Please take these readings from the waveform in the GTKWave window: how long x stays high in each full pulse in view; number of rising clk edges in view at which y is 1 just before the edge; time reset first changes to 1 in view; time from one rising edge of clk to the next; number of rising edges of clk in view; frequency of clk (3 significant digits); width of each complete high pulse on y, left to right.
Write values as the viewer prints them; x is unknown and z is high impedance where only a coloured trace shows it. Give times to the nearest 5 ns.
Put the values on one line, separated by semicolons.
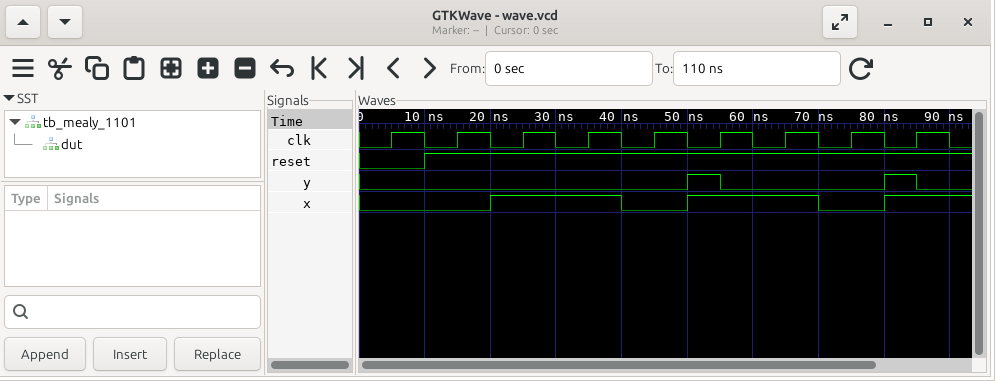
20 ns, 20 ns; 2; 10 ns; 10 ns; 9; 100 MHz; 5 ns, 5 ns
